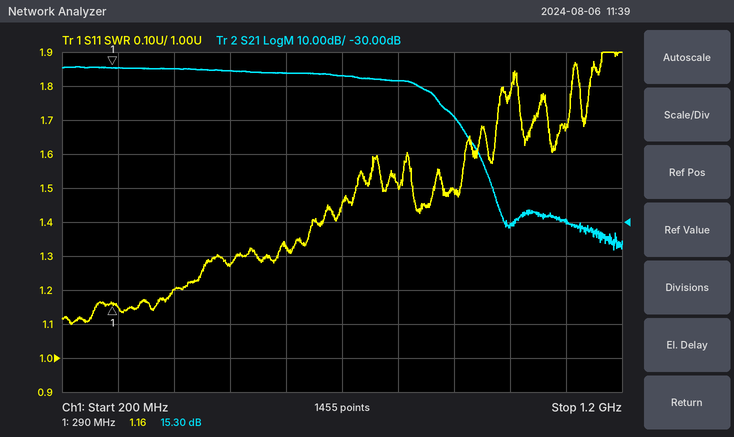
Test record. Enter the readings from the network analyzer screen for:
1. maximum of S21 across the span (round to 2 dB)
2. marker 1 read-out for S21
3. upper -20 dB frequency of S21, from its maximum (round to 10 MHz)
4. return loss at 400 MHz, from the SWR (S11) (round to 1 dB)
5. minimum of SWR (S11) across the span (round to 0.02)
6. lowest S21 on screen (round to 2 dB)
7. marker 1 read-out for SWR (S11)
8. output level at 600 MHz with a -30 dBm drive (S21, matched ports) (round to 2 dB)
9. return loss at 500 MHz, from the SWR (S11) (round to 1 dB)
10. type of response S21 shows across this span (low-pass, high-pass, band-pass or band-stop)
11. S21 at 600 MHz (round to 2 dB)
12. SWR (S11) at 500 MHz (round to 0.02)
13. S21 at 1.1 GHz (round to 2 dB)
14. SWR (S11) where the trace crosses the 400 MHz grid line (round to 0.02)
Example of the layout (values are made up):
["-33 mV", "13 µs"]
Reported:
["16 dB", "15.30 dB", "920 MHz", "21 dB", "1.10", "-38 dB", "1.16", "-16 dBm", "18 dB", "low-pass", "14 dB", "1.28", "-30 dB", "1.20"]
